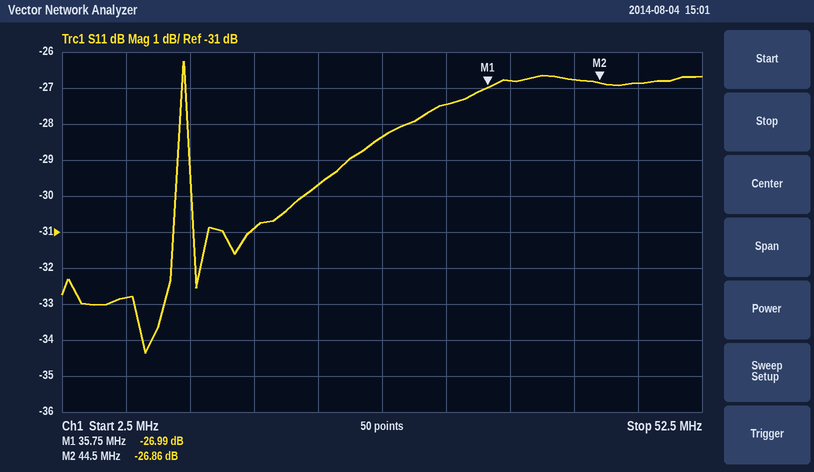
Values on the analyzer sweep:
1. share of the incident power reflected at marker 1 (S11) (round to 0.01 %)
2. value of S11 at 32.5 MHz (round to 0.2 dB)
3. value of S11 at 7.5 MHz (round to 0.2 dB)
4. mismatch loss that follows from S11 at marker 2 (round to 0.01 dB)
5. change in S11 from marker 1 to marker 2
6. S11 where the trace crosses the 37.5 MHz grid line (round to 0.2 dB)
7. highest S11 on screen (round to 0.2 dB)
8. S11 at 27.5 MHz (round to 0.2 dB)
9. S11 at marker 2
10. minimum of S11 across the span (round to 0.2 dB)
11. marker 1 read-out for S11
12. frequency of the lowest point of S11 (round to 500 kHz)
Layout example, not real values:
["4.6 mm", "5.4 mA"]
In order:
["0.20 %", "-27.4 dB", "-32.8 dB", "0.01 dB", "0.13 dB", "-26.8 dB", "-26.2 dB", "-28.4 dB", "-26.86 dB", "-34.4 dB", "-26.99 dB", "9.0 MHz"]
